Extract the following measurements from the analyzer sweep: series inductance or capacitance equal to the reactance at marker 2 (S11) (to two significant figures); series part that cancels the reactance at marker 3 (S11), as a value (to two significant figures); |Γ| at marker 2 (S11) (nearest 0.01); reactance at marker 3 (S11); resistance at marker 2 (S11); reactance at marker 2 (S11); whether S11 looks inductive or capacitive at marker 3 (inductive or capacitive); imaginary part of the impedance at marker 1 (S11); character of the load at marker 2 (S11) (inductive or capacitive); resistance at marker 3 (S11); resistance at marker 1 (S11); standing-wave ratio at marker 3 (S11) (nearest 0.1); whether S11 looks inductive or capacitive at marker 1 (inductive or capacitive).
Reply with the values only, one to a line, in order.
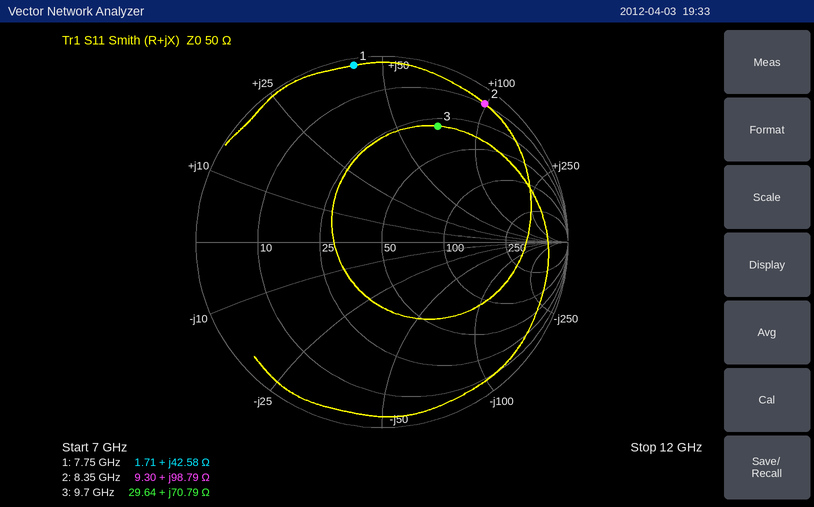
1.9 nH
230 fF
0.93
+70.79 Ω
9.30 Ω
+98.79 Ω
inductive
+42.58 Ω
inductive
29.64 Ω
1.71 Ω
5.5
inductive
